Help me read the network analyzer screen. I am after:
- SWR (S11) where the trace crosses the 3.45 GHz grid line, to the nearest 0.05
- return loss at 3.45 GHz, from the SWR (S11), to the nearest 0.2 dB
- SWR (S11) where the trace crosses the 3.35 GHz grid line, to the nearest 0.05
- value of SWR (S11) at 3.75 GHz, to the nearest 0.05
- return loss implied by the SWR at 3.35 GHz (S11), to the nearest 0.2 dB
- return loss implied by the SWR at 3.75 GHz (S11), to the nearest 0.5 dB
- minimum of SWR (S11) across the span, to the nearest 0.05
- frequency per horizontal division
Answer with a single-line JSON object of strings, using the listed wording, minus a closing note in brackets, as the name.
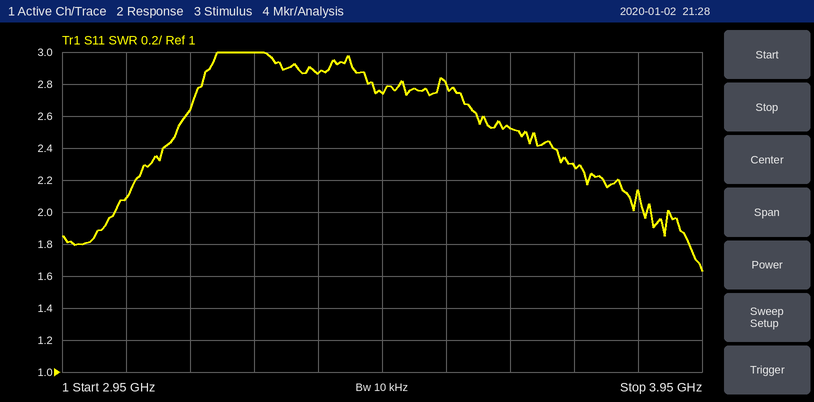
{"SWR (S11) where the trace crosses the 3.45 GHz grid line, to the nearest 0.05": "2.75", "return loss at 3.45 GHz, from the SWR (S11), to the nearest 0.2 dB": "6.6 dB", "SWR (S11) where the trace crosses the 3.35 GHz grid line, to the nearest 0.05": "2.85", "value of SWR (S11) at 3.75 GHz, to the nearest 0.05": "2.30", "return loss implied by the SWR at 3.35 GHz (S11), to the nearest 0.2 dB": "6.4 dB", "return loss implied by the SWR at 3.75 GHz (S11), to the nearest 0.5 dB": "8.0 dB", "minimum of SWR (S11) across the span, to the nearest 0.05": "1.65", "frequency per horizontal division": "100 MHz"}
